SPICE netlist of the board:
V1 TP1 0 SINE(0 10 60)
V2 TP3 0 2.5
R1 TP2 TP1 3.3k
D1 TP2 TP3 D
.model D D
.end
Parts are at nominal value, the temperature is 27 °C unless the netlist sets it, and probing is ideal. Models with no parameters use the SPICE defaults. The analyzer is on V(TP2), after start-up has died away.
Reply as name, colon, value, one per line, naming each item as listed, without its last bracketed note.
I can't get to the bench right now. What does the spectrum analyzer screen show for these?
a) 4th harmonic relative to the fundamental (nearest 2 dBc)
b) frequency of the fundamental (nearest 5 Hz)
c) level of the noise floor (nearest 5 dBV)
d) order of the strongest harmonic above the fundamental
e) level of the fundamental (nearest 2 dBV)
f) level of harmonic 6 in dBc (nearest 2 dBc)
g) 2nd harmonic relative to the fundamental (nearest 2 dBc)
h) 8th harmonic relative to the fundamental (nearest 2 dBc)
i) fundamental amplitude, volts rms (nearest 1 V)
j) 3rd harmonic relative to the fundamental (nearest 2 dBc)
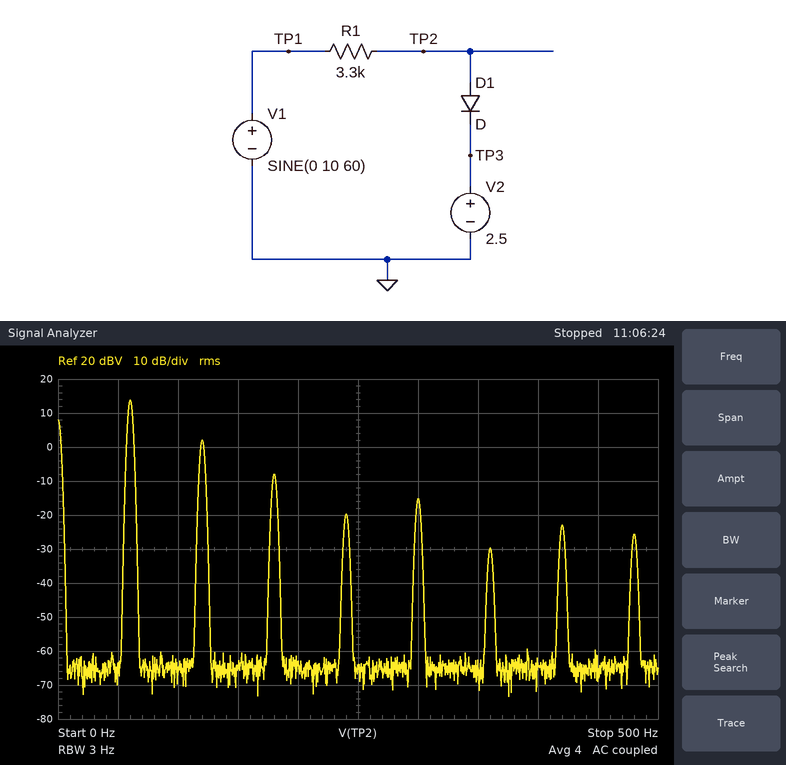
4th harmonic relative to the fundamental: -34 dBc
frequency of the fundamental: 60 Hz
level of the noise floor: -65 dBV
order of the strongest harmonic above the fundamental: 2
level of the fundamental: 14 dBV
level of harmonic 6 in dBc: -44 dBc
2nd harmonic relative to the fundamental: -12 dBc
8th harmonic relative to the fundamental: -40 dBc
fundamental amplitude, volts rms: 5 V
3rd harmonic relative to the fundamental: -22 dBc
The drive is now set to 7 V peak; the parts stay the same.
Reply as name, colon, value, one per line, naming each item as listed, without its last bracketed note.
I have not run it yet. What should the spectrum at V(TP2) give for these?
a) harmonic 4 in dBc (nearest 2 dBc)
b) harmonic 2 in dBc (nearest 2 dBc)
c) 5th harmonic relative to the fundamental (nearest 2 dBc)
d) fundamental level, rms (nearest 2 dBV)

harmonic 4 in dBc: -42 dBc
harmonic 2 in dBc: -14 dBc
5th harmonic relative to the fundamental: -32 dBc
fundamental level, rms: 12 dBV
